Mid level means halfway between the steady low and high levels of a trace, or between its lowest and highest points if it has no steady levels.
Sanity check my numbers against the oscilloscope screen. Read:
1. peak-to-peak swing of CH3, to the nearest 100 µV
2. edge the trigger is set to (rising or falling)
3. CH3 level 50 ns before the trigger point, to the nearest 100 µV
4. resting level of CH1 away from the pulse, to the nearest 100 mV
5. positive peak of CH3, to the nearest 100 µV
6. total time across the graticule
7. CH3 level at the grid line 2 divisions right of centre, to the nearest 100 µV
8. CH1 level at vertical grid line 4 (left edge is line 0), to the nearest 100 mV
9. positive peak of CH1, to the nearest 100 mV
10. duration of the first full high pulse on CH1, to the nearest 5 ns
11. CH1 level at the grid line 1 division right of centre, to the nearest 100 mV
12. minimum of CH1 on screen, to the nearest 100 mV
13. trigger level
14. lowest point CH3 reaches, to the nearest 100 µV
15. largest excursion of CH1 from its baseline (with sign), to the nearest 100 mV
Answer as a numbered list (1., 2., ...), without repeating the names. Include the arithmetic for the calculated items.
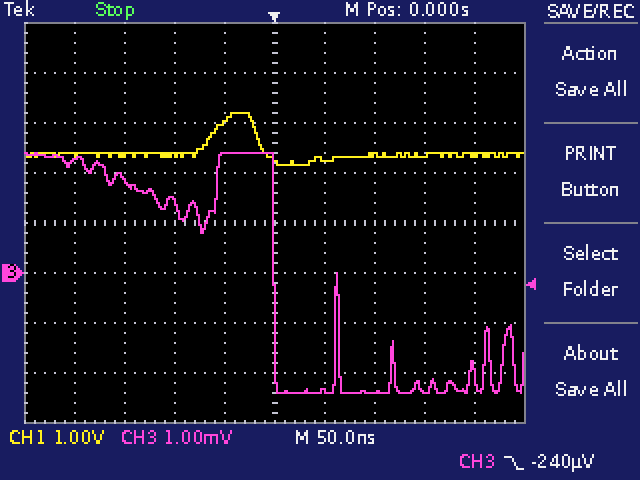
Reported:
1. 2.4 mV − (-2.4 mV) = 4.8 mV
2. falling
3. 2.4 mV
4. 2.4 V
5. 2.4 mV
6. 500 ns
7. -2.4 mV
8. 3.0 V
9. 3.2 V
10. 50 ns
11. 2.3 V
12. 2.2 V
13. -240 µV
14. -2.4 mV
15. 3.2 V − (2.4 V) = +800 mV
